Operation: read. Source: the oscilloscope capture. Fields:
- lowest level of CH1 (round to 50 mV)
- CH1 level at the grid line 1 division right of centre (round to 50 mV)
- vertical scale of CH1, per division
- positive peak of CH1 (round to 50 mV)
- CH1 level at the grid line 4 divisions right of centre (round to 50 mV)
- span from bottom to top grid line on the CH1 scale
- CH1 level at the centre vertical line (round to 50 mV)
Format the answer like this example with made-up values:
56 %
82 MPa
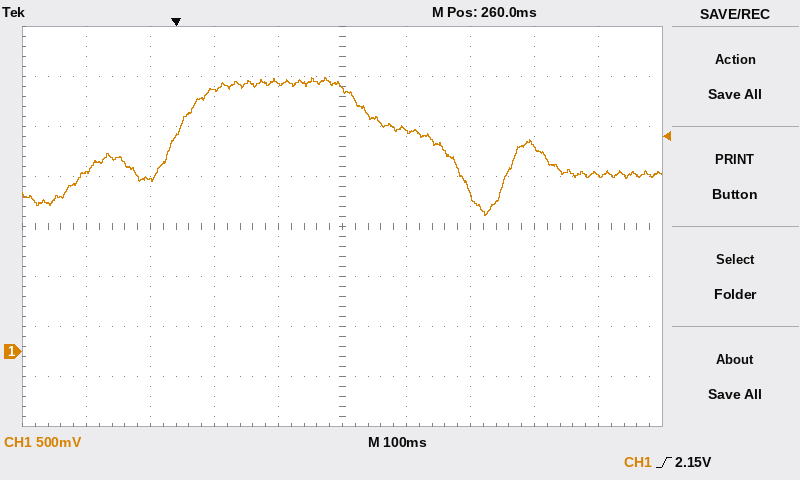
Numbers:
1.35 V
2.20 V
500 mV
2.75 V
1.75 V
4 V
2.65 V
